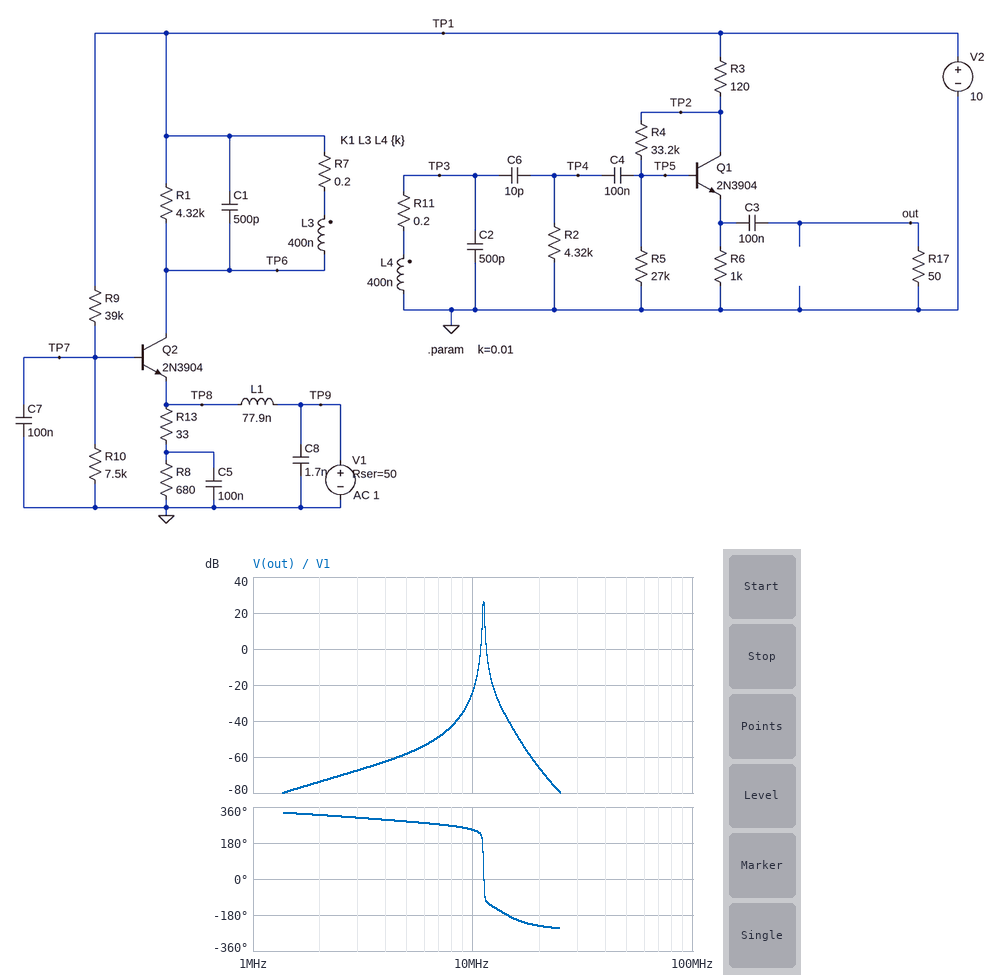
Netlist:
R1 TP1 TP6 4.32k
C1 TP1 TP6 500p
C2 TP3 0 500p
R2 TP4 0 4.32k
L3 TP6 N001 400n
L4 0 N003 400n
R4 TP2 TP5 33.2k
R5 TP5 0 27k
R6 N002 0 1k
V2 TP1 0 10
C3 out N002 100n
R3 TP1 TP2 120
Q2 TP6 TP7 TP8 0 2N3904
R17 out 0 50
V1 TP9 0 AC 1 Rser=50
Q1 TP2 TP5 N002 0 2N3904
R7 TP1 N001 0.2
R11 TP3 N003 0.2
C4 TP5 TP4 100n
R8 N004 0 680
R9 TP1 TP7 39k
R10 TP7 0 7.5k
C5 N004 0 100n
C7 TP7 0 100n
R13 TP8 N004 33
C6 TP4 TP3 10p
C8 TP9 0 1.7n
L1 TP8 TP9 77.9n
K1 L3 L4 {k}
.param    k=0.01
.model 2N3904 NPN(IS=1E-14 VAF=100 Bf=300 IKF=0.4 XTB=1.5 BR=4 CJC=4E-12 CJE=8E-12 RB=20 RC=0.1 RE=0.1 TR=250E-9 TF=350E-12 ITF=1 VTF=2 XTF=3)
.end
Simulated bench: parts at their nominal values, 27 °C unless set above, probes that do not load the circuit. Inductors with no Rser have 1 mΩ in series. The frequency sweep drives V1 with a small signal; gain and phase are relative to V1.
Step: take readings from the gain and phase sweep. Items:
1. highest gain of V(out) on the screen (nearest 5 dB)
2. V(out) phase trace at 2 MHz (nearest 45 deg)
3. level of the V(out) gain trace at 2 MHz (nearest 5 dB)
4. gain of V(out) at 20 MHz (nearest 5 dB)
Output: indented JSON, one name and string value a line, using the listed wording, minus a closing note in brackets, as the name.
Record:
{
  "highest gain of V(out) on the screen": "25 dB",
  "V(out) phase trace at 2 MHz": "315 deg",
  "level of the V(out) gain trace at 2 MHz": "-75 dB",
  "gain of V(out) at 20 MHz": "-65 dB"
}
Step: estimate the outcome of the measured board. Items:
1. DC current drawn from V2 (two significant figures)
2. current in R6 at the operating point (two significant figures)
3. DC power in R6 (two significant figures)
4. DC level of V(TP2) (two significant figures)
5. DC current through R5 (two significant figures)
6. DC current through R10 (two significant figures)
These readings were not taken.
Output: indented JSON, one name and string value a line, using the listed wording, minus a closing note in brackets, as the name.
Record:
{
  "DC current drawn from V2": "17 mA",
  "current in R6 at the operating point": "3.4 mA",
  "DC power in R6": "12 mW",
  "DC level of V(TP2)": "9.6 V",
  "DC current through R5": "150 µA",
  "DC current through R10": "180 µA"
}
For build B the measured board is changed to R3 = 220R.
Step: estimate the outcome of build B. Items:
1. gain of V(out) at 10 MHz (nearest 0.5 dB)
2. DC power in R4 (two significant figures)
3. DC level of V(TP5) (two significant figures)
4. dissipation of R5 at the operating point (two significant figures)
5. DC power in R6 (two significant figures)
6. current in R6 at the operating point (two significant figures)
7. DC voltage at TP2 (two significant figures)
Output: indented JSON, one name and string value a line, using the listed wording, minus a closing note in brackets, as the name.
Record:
{
  "gain of V(out) at 10 MHz": "-24.5 dB",
  "DC power in R4": "830 µW",
  "DC level of V(TP5)": "4.0 V",
  "dissipation of R5 at the operating point": "590 µW",
  "DC power in R6": "11 mW",
  "current in R6 at the operating point": "3.3 mA",
  "DC voltage at TP2": "9.2 V"
}
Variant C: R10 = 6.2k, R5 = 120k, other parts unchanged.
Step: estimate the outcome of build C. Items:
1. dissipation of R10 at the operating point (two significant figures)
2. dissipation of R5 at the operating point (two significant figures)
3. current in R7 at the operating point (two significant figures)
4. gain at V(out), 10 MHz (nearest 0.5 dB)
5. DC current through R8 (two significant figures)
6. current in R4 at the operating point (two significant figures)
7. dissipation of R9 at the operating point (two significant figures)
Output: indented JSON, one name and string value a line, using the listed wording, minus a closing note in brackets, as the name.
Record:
{
  "dissipation of R10 at the operating point": "230 µW",
  "dissipation of R5 at the operating point": "380 µW",
  "current in R7 at the operating point": "10 mA",
  "gain at V(out), 10 MHz": "-24.0 dB",
  "DC current through R8": "680 µA",
  "current in R4 at the operating point": "76 µA",
  "dissipation of R9 at the operating point": "2.0 mW"
}
